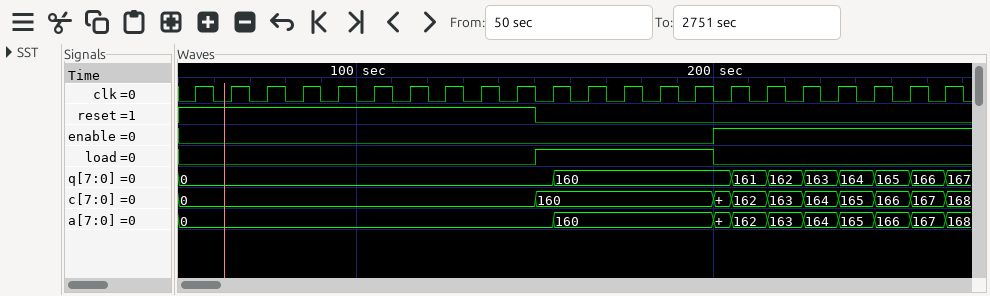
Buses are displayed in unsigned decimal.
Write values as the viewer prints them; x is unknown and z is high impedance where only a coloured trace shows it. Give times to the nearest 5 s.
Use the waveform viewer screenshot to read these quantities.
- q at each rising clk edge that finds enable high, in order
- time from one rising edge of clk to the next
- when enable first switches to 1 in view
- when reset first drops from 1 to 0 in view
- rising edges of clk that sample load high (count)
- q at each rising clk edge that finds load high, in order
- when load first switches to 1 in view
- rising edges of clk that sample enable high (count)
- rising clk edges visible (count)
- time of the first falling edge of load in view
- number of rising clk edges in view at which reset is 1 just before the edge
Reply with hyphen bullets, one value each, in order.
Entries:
- 160, 161, 162, 163, 164, 165, 166
- 10 s
- 200 s
- 150 s
- 5
- 0, 160, 160, 160, 160
- 150 s
- 7
- 22
- 200 s
- 10
